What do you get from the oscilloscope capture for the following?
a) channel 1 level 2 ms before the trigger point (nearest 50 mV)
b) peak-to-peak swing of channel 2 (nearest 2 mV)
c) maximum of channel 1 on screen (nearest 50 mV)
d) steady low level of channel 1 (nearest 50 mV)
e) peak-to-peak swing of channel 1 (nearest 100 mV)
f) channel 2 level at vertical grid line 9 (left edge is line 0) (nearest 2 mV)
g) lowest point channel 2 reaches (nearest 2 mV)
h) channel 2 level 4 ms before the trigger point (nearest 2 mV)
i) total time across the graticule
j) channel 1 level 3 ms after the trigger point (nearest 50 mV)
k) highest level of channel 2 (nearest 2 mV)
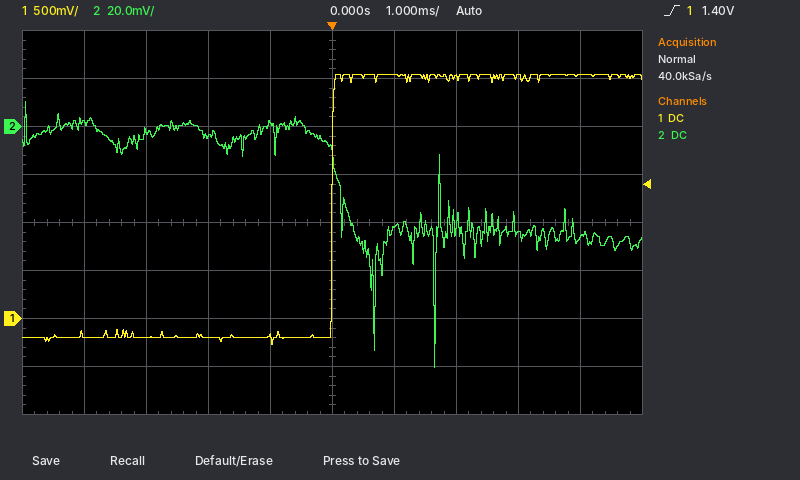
-200 mV
110 mV
2.55 V
-200 mV
2.80 V
-46 mV
-100 mV
2 mV
10 ms
2.50 V
10 mV
